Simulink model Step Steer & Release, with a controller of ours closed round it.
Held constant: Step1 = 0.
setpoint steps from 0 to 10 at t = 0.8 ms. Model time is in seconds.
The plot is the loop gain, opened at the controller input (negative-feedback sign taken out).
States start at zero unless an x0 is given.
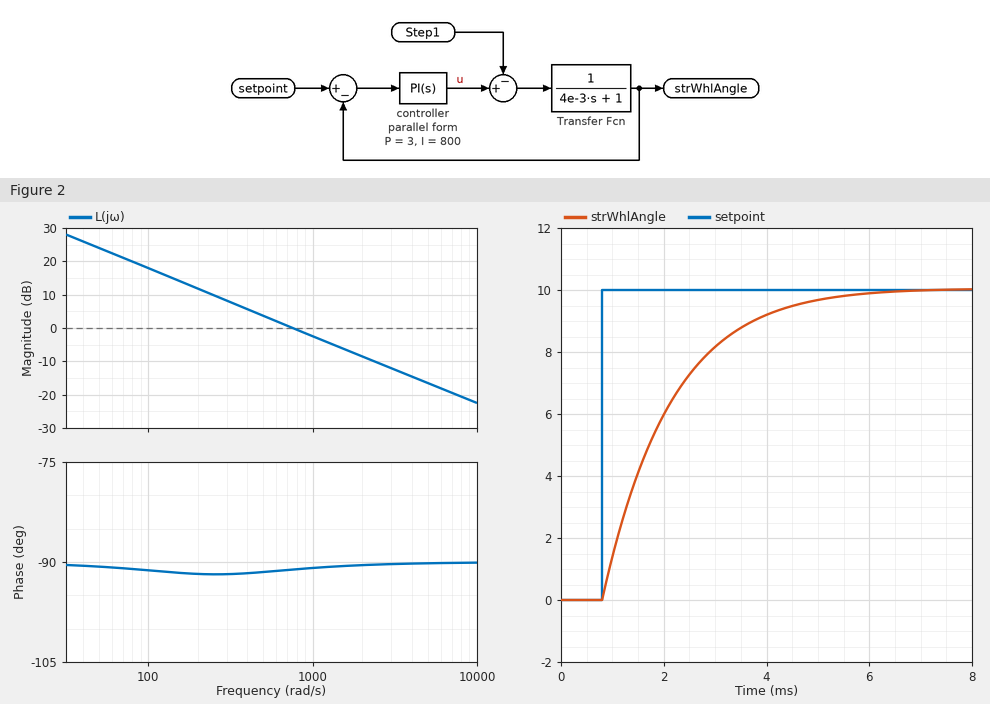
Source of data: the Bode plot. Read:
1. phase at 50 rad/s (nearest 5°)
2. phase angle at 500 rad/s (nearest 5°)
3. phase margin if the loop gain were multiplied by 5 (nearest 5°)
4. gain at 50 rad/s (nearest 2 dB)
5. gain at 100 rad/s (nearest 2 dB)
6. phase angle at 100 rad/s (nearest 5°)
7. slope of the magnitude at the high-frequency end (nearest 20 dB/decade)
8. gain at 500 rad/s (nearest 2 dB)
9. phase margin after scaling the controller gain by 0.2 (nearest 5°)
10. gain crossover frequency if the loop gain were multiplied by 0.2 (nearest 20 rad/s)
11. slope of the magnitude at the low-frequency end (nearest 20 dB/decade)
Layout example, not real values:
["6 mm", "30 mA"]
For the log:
["-90°", "-90°", "90°", "24 dB", "18 dB", "-90°", "-20 dB/decade", "4 dB", "90°", "160 rad/s", "-20 dB/decade"]
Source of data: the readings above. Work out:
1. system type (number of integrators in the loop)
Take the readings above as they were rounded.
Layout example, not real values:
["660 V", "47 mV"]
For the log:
["1"]
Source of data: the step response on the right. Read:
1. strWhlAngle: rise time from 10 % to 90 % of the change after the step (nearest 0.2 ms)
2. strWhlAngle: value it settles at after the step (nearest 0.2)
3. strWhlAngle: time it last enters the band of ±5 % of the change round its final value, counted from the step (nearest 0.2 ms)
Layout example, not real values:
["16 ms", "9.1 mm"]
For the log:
["2.8 ms", "10.0", "3.8 ms"]
